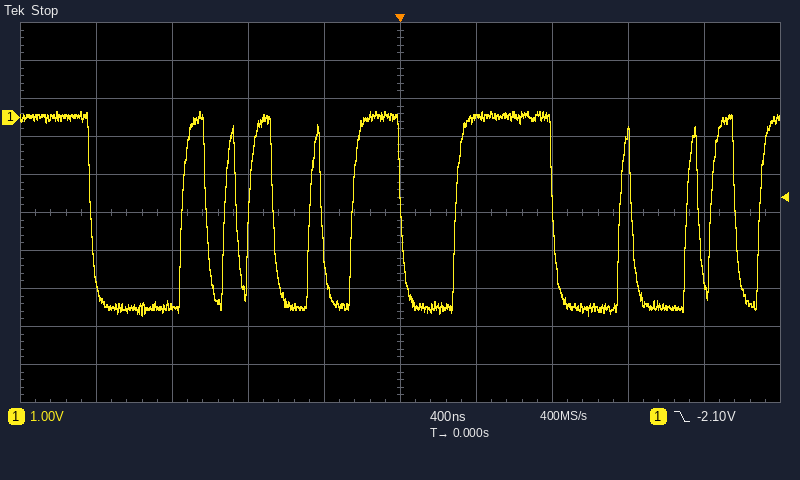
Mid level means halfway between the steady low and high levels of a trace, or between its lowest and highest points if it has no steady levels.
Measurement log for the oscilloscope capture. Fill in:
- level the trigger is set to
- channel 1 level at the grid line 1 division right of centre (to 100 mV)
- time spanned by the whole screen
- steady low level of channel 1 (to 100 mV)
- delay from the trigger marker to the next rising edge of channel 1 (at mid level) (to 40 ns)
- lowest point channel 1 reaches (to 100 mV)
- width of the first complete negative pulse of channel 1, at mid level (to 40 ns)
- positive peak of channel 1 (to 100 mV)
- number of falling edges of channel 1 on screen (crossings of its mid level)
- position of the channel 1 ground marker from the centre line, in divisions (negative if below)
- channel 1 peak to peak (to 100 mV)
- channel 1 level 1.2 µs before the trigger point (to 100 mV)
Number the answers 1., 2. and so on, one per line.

1. -2.10 V
2. 0.0 V
3. 4 µs
4. -5.0 V
5. 280 ns
6. -5.2 V
7. 480 ns
8. 200 mV
9. 10
10. +2.5 div
11. 5.4 V
12. -5.0 V
